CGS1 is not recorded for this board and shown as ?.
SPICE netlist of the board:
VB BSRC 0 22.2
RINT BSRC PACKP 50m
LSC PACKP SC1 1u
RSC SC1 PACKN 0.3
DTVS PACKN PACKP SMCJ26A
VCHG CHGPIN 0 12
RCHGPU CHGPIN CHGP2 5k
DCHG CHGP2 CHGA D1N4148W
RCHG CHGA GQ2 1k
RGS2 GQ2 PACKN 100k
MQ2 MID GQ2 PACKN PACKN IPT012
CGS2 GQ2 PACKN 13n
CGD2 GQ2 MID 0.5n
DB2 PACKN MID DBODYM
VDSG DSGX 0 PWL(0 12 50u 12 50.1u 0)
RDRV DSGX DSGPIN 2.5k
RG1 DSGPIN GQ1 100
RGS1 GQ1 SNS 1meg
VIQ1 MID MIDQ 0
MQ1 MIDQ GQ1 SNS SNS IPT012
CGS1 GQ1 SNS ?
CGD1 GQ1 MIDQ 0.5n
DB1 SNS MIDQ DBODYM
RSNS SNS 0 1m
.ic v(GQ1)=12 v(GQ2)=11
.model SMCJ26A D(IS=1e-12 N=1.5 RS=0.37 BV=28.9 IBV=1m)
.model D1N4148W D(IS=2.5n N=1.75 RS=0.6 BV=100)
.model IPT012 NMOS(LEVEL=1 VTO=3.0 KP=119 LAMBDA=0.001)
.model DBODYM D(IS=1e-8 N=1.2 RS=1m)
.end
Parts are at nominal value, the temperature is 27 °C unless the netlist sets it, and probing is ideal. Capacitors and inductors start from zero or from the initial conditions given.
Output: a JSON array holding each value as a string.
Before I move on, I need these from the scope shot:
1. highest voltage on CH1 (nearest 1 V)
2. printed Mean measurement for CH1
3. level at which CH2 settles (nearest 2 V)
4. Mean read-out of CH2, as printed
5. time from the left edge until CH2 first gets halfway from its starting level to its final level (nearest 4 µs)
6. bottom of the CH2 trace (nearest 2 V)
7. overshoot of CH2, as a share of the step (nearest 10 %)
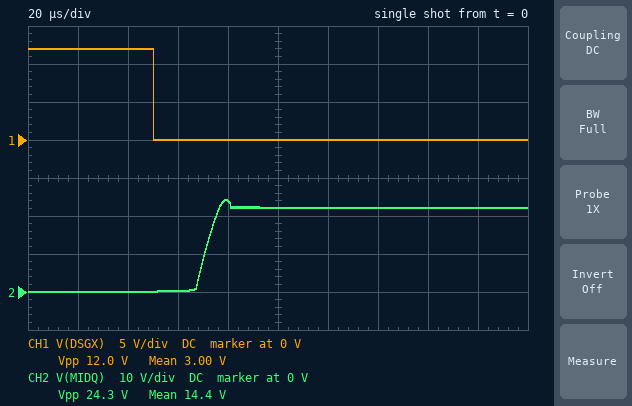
["12 V", "3.00 V", "22 V", "14.4 V", "72 µs", "0 V", "10 %"]
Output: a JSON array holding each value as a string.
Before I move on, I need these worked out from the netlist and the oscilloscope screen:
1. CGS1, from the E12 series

["5.6 nF"]
